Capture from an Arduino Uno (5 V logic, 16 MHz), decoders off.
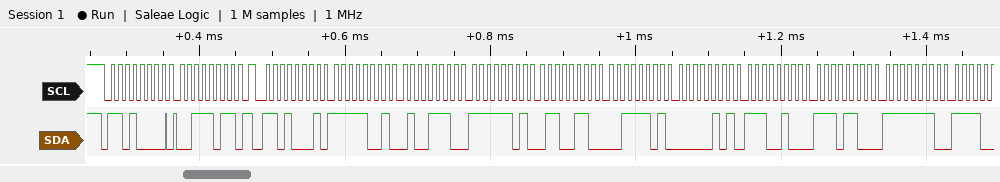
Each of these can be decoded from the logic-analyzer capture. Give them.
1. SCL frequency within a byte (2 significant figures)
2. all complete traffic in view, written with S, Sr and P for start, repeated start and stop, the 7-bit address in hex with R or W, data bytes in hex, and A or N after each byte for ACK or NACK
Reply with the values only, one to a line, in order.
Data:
100 kHz
S 68W A 3B A Sr 68R A F9 A 4E A FD A 66 A 3D A 05 A E4 A EC A FE A
